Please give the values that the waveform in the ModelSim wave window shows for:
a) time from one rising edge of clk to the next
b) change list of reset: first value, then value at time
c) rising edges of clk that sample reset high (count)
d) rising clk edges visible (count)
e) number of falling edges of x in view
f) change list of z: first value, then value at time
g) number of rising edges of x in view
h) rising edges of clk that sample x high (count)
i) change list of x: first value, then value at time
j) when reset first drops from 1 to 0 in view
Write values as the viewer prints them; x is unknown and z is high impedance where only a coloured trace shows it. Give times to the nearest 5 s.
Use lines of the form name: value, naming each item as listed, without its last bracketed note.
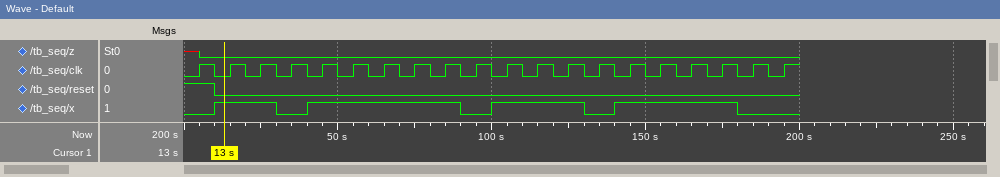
time from one rising edge of clk to the next: 10 s
change list of reset: first value, then value at time: 1, 0 at 10 s
rising edges of clk that sample reset high: 1
rising clk edges visible: 20
number of falling edges of x in view: 4
change list of z: first value, then value at time: x, 0 at 5 s
number of rising edges of x in view: 4
rising edges of clk that sample x high: 14
change list of x: first value, then value at time: 0, 1 at 10 s, 0 at 30 s, 1 at 40 s, 0 at 90 s, 1 at 100 s, 0 at 130 s, 1 at 140 s, 0 at 180 s
when reset first drops from 1 to 0 in view: 10 s
